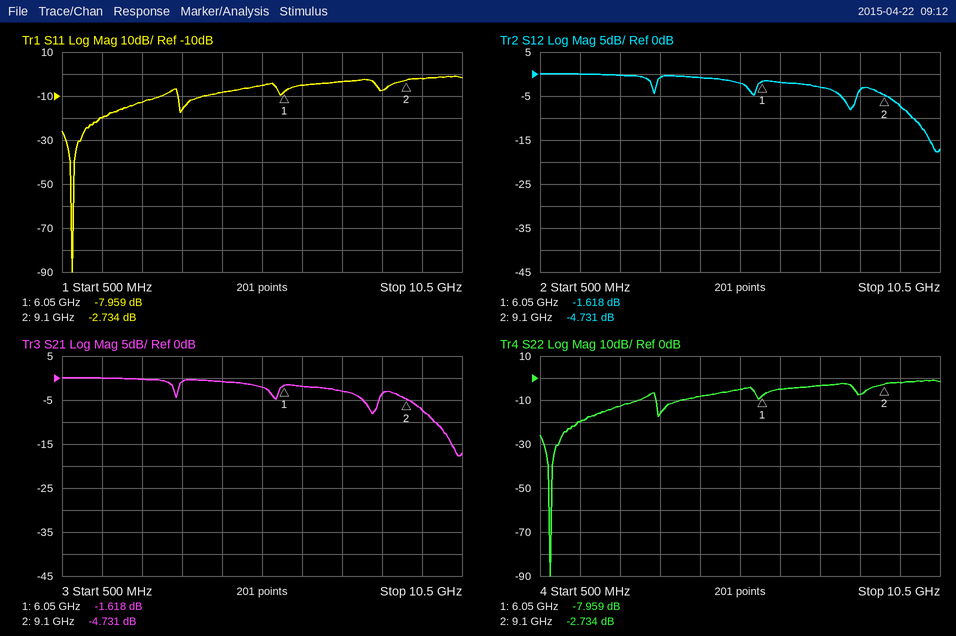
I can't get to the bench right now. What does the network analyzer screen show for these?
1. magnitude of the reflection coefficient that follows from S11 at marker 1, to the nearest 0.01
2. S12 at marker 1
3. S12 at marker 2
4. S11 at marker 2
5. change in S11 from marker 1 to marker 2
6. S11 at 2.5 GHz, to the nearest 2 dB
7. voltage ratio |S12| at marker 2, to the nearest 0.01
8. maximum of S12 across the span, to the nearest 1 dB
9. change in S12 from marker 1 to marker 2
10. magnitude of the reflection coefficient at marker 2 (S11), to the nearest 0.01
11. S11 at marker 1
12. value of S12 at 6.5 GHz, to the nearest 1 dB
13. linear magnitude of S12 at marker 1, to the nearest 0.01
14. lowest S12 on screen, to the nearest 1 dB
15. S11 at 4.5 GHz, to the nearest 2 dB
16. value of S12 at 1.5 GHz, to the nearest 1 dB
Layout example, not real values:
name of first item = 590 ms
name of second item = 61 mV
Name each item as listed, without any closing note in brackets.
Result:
magnitude of the reflection coefficient that follows from S11 at marker 1, to the nearest 0.01 = 0.40
S12 at marker 1 = -1.618 dB
S12 at marker 2 = -4.731 dB
S11 at marker 2 = -2.734 dB
change in S11 from marker 1 to marker 2 = 5.225 dB
S11 at 2.5 GHz, to the nearest 2 dB = -12 dB
voltage ratio |S12| at marker 2, to the nearest 0.01 = 0.58
maximum of S12 across the span, to the nearest 1 dB = 0 dB
change in S12 from marker 1 to marker 2 = -3.113 dB
magnitude of the reflection coefficient at marker 2 (S11), to the nearest 0.01 = 0.73
S11 at marker 1 = -7.959 dB
value of S12 at 6.5 GHz, to the nearest 1 dB = -2 dB
linear magnitude of S12 at marker 1, to the nearest 0.01 = 0.83
lowest S12 on screen, to the nearest 1 dB = -18 dB
S11 at 4.5 GHz, to the nearest 2 dB = -8 dB
value of S12 at 1.5 GHz, to the nearest 1 dB = 0 dB
